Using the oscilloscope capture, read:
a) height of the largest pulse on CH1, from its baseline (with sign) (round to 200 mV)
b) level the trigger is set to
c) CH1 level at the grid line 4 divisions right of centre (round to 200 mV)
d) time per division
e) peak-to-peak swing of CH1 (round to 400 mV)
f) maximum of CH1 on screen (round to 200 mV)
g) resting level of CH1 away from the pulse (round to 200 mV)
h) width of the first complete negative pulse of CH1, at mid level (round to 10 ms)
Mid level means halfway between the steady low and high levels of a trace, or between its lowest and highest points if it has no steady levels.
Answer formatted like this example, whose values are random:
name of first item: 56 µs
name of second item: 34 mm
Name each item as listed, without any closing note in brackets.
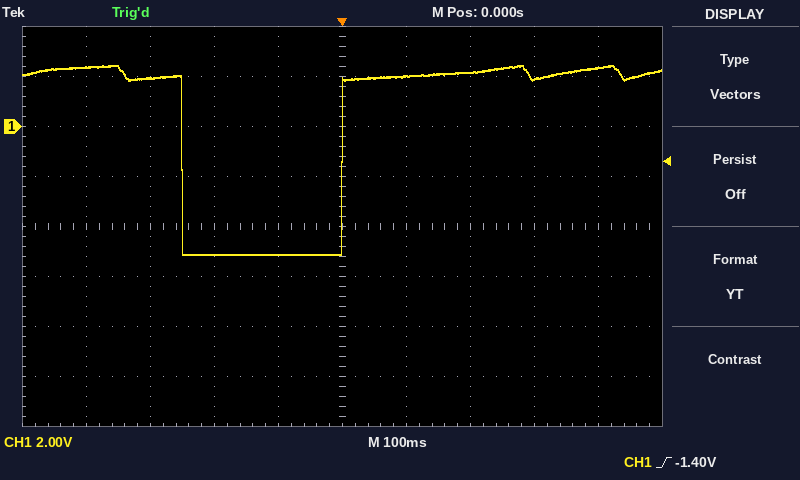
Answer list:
height of the largest pulse on CH1, from its baseline (with sign): -7.2 V
level the trigger is set to: -1.40 V
CH1 level at the grid line 4 divisions right of centre: 2.4 V
time per division: 100 ms
peak-to-peak swing of CH1: 7.6 V
maximum of CH1 on screen: 2.4 V
resting level of CH1 away from the pulse: 2.0 V
width of the first complete negative pulse of CH1, at mid level: 250 ms
